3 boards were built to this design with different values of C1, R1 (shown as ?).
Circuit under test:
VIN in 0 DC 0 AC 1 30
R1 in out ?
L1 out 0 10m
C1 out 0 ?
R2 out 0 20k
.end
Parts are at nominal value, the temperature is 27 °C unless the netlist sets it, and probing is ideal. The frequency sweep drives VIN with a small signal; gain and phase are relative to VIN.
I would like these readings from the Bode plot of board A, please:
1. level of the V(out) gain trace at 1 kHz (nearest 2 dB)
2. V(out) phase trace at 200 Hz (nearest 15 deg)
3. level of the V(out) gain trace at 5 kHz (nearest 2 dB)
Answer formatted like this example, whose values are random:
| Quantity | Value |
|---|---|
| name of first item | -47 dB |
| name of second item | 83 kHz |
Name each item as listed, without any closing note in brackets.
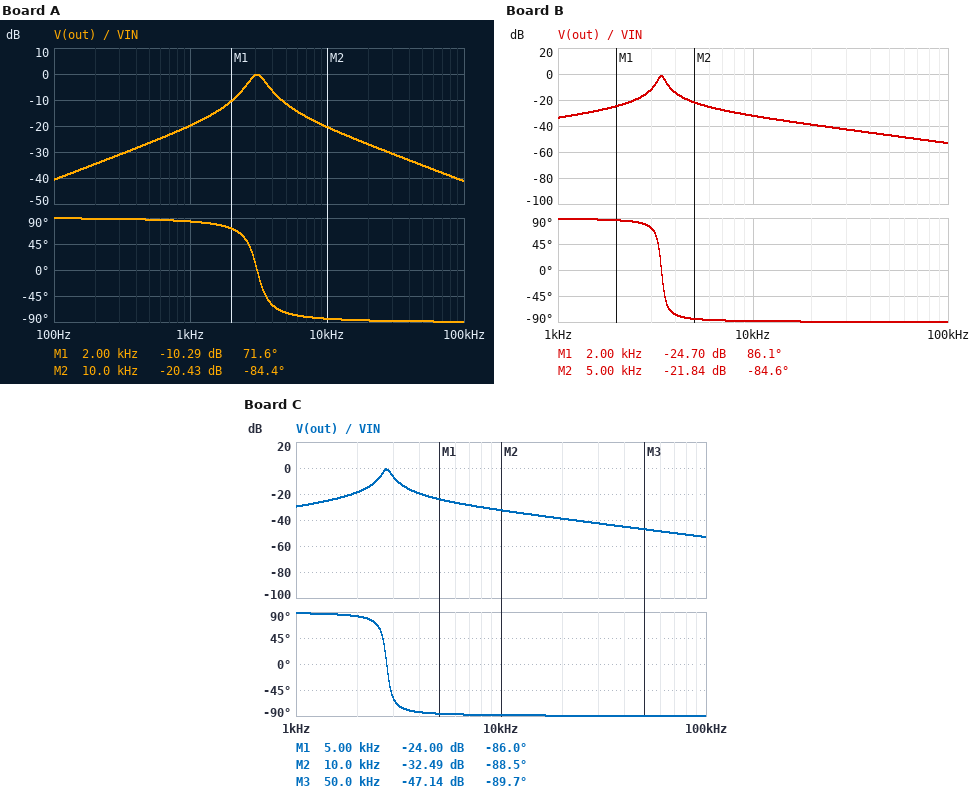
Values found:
| Quantity | Value |
|---|---|
| level of the V(out) gain trace at 1 kHz | -20 dB |
| V(out) phase trace at 200 Hz | 90 deg |
| level of the V(out) gain trace at 5 kHz | -12 dB |
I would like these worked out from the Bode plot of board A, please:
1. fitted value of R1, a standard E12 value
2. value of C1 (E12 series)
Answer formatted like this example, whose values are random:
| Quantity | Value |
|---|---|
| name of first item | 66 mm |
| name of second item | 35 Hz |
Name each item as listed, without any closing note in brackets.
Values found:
| Quantity | Value |
|---|---|
| fitted value of R1, a standard E12 value | 680 Ω |
| value of C1 | 270 nF |
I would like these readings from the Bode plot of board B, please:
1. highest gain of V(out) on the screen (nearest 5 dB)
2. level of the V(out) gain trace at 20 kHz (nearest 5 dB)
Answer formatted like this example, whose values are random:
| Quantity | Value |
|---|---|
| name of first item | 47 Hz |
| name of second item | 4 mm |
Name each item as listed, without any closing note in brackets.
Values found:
| Quantity | Value |
|---|---|
| highest gain of V(out) on the screen | 0 dB |
| level of the V(out) gain trace at 20 kHz | -40 dB |
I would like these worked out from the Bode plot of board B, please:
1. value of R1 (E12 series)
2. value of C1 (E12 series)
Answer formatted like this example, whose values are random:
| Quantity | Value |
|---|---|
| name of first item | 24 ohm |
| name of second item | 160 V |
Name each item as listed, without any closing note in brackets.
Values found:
| Quantity | Value |
|---|---|
| value of R1 | 3.3 kΩ |
| value of C1 | 220 nF |
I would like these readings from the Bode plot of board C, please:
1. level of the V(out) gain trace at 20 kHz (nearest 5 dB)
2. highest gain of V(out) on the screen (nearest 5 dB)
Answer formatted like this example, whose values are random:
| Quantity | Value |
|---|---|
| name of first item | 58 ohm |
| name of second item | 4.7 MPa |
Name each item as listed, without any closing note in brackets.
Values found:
| Quantity | Value |
|---|---|
| level of the V(out) gain trace at 20 kHz | -40 dB |
| highest gain of V(out) on the screen | 0 dB |
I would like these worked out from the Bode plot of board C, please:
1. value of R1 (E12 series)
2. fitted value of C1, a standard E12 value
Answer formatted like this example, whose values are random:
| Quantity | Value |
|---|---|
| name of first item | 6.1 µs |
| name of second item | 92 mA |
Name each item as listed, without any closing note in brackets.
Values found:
| Quantity | Value |
|---|---|
| value of R1 | 2.2 kΩ |
| fitted value of C1, a standard E12 value | 330 nF |
